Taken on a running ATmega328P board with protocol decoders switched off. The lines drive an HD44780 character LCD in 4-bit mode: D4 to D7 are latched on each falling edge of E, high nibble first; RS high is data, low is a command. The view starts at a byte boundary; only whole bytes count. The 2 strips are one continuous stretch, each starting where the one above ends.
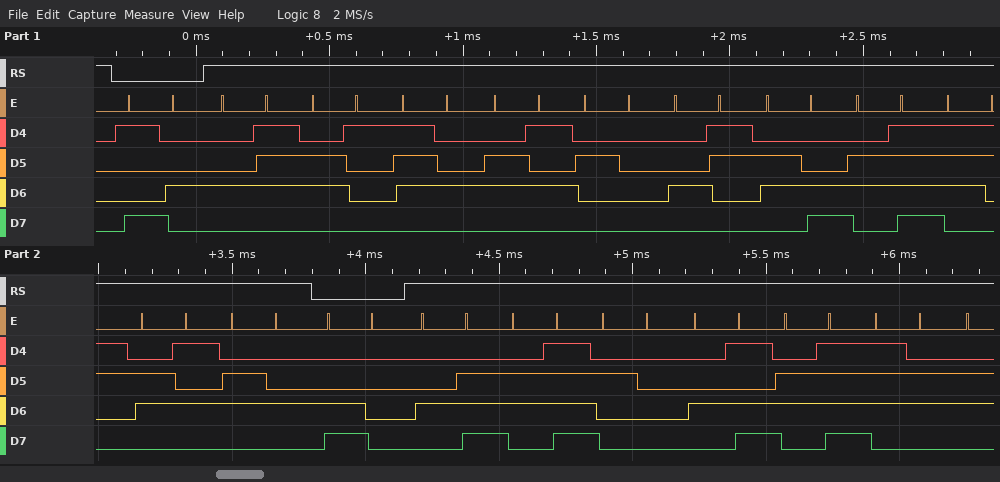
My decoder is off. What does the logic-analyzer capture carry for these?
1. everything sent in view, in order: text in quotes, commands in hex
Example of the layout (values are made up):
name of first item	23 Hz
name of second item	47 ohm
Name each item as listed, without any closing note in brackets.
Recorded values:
everything sent in view, in order: text in quotes, commands in hex	0x94 "Gate Closed" 0xC0 "No Mov"
